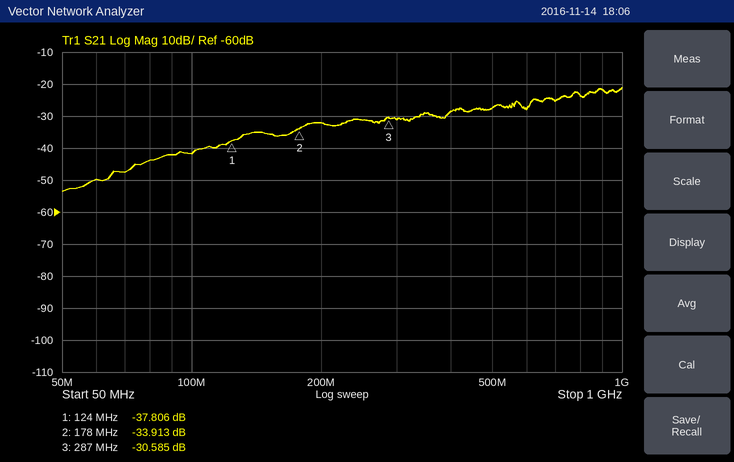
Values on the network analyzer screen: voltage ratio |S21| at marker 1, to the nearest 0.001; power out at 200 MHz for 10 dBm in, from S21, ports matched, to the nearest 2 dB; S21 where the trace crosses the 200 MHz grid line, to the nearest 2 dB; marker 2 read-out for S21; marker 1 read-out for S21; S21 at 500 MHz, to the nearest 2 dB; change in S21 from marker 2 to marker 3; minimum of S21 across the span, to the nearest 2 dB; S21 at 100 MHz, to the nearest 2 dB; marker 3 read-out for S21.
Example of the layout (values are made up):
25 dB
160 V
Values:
0.013
-22 dBm
-32 dB
-33.913 dB
-37.806 dB
-28 dB
3.328 dB
-54 dB
-42 dB
-30.585 dB
